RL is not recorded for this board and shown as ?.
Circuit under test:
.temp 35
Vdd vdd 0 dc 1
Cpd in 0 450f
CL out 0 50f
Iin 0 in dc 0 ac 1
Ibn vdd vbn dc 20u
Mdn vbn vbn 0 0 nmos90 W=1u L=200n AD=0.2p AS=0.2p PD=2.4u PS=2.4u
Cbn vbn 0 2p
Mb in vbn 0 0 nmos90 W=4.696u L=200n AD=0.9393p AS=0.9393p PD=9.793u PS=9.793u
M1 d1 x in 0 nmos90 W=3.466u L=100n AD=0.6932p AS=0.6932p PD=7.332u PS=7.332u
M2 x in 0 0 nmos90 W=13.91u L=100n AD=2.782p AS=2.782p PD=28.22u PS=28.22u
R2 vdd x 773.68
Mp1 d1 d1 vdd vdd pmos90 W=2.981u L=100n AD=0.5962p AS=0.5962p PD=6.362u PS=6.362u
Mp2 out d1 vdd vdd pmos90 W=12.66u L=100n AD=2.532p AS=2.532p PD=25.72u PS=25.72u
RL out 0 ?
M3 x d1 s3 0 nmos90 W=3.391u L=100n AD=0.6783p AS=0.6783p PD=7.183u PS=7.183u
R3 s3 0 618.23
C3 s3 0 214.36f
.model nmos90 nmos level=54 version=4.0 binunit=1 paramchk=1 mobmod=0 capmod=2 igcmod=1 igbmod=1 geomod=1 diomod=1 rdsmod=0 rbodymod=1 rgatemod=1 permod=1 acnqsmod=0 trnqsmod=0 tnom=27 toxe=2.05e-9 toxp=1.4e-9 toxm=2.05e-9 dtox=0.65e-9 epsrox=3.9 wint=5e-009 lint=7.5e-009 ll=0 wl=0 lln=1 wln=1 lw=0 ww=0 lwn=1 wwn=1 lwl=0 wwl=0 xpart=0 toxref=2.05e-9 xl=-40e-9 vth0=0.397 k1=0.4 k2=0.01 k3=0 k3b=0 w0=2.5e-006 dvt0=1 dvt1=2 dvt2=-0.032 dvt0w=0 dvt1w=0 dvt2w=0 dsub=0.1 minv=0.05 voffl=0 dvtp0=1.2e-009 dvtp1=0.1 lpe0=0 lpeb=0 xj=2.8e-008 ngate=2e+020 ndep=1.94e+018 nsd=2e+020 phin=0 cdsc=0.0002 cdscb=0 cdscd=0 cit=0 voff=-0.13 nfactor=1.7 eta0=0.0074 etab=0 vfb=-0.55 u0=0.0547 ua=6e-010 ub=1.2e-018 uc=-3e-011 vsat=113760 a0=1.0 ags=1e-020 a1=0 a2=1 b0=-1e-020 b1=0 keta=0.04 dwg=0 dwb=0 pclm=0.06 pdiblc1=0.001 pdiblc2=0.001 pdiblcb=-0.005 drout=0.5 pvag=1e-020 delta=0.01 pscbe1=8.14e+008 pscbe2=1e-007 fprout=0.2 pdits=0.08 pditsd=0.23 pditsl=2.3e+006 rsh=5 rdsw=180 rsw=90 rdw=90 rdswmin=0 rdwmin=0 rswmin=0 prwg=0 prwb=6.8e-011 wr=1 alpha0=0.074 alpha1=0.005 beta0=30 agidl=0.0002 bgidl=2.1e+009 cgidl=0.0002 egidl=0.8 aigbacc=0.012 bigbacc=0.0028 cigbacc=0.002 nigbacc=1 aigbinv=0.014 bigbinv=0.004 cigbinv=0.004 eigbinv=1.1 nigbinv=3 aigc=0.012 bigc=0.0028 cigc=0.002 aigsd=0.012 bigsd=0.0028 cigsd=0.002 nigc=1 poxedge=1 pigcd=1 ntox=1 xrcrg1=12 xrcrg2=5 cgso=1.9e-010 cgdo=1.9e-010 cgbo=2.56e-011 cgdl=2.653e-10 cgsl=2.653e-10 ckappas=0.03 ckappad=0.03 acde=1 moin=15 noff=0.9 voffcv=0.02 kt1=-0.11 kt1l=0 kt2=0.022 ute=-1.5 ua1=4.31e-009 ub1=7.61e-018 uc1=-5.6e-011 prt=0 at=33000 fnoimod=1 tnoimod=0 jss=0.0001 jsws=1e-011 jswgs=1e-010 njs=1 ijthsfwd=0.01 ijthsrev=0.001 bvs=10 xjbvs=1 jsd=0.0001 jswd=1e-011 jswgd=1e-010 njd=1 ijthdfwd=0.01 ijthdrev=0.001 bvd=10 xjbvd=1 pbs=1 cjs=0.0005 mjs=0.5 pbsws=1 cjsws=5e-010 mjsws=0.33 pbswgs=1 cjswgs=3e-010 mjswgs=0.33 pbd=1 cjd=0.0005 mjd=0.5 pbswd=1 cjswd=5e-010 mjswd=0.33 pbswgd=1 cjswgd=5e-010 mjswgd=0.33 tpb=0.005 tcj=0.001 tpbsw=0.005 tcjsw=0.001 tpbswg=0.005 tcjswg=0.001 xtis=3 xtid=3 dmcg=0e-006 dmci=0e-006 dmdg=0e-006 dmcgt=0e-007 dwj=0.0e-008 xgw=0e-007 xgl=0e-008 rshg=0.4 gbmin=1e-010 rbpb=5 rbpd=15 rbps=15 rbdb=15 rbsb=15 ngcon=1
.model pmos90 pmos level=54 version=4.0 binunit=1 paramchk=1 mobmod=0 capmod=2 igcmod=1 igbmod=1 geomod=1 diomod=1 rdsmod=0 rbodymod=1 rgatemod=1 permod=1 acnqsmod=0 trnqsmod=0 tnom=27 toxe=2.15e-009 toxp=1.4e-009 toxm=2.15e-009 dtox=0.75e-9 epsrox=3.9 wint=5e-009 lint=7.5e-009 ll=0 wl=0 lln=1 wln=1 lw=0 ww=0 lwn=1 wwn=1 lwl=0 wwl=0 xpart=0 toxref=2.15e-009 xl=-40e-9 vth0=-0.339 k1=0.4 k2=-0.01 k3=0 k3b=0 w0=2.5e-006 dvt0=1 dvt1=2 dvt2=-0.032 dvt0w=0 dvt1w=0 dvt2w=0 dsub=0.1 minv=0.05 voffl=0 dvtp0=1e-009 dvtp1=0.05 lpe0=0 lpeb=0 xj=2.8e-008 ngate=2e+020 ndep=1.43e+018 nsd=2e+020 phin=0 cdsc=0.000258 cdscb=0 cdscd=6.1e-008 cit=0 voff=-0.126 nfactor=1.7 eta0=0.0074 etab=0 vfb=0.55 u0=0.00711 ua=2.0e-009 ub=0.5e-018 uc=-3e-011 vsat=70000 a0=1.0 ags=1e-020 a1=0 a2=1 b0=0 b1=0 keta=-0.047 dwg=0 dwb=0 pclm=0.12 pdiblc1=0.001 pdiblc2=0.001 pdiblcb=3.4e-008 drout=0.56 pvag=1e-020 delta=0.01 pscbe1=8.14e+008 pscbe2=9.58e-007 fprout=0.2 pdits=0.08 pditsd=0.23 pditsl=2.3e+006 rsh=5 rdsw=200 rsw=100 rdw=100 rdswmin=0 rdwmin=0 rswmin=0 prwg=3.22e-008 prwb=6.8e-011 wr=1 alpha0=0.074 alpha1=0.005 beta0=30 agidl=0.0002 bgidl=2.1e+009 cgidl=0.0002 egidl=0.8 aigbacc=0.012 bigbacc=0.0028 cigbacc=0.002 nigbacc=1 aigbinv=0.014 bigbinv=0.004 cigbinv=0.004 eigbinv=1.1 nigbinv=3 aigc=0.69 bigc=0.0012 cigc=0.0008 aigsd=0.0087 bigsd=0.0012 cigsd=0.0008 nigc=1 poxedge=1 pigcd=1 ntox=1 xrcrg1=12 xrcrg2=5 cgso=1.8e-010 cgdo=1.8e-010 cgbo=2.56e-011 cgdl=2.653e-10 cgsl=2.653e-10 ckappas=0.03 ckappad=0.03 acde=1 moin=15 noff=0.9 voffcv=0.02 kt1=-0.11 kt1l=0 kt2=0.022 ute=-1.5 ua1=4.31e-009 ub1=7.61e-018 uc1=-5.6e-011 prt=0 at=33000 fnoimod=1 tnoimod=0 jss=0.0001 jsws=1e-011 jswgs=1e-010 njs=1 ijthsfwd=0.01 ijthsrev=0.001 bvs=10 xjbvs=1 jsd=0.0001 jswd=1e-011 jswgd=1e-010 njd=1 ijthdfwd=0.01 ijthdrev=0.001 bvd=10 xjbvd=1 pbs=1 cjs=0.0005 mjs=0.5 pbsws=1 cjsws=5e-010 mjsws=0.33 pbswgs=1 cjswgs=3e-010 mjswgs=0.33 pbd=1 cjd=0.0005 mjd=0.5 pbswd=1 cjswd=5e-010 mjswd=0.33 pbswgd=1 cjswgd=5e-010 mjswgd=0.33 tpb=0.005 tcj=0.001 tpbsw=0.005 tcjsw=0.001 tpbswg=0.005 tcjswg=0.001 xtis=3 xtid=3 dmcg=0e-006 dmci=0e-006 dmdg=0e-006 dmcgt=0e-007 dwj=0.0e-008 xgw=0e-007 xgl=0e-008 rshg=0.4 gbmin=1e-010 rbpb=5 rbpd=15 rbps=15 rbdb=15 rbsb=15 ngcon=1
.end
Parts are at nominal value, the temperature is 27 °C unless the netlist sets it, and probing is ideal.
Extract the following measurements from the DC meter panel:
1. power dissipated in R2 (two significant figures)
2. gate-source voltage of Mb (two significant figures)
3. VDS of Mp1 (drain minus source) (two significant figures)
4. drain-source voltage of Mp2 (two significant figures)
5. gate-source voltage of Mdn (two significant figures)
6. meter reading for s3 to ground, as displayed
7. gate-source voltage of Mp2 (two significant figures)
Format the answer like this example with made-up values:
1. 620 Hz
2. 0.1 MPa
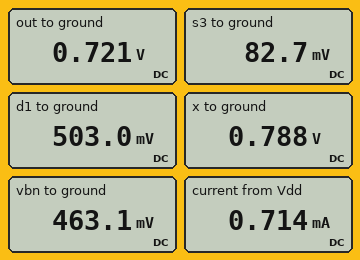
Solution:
1. 58 µW
2. 460 mV
3. -500 mV
4. -280 mV
5. 460 mV
6. 82.7 mV
7. -500 mV
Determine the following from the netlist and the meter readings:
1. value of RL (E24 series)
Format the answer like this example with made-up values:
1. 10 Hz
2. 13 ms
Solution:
1. 2.2 kΩ
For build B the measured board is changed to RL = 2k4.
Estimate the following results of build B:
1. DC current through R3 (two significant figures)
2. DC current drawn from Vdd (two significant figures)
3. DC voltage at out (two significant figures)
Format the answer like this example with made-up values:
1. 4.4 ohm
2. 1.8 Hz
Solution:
1. 130 µA
2. 700 µA
3. 760 mV
